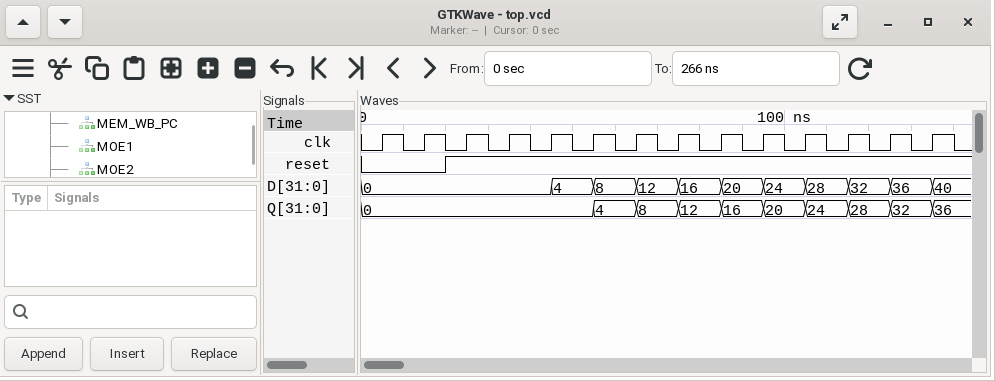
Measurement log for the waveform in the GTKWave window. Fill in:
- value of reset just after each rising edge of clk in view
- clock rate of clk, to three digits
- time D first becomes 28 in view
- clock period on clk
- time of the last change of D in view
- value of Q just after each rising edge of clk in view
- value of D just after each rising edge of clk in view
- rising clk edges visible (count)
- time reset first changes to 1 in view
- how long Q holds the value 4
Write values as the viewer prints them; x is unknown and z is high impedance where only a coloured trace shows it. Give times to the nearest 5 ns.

0 0 1 1 1 1 1 1 1 1 1 1 1 1
100 MHz
105 ns
10 ns
135 ns
0, 0, 0, 0, 0, 4, 8, 12, 16, 20, 24, 28, 32, 36
0, 0, 0, 0, 4, 8, 12, 16, 20, 24, 28, 32, 36, 40
14
20 ns
10 ns
